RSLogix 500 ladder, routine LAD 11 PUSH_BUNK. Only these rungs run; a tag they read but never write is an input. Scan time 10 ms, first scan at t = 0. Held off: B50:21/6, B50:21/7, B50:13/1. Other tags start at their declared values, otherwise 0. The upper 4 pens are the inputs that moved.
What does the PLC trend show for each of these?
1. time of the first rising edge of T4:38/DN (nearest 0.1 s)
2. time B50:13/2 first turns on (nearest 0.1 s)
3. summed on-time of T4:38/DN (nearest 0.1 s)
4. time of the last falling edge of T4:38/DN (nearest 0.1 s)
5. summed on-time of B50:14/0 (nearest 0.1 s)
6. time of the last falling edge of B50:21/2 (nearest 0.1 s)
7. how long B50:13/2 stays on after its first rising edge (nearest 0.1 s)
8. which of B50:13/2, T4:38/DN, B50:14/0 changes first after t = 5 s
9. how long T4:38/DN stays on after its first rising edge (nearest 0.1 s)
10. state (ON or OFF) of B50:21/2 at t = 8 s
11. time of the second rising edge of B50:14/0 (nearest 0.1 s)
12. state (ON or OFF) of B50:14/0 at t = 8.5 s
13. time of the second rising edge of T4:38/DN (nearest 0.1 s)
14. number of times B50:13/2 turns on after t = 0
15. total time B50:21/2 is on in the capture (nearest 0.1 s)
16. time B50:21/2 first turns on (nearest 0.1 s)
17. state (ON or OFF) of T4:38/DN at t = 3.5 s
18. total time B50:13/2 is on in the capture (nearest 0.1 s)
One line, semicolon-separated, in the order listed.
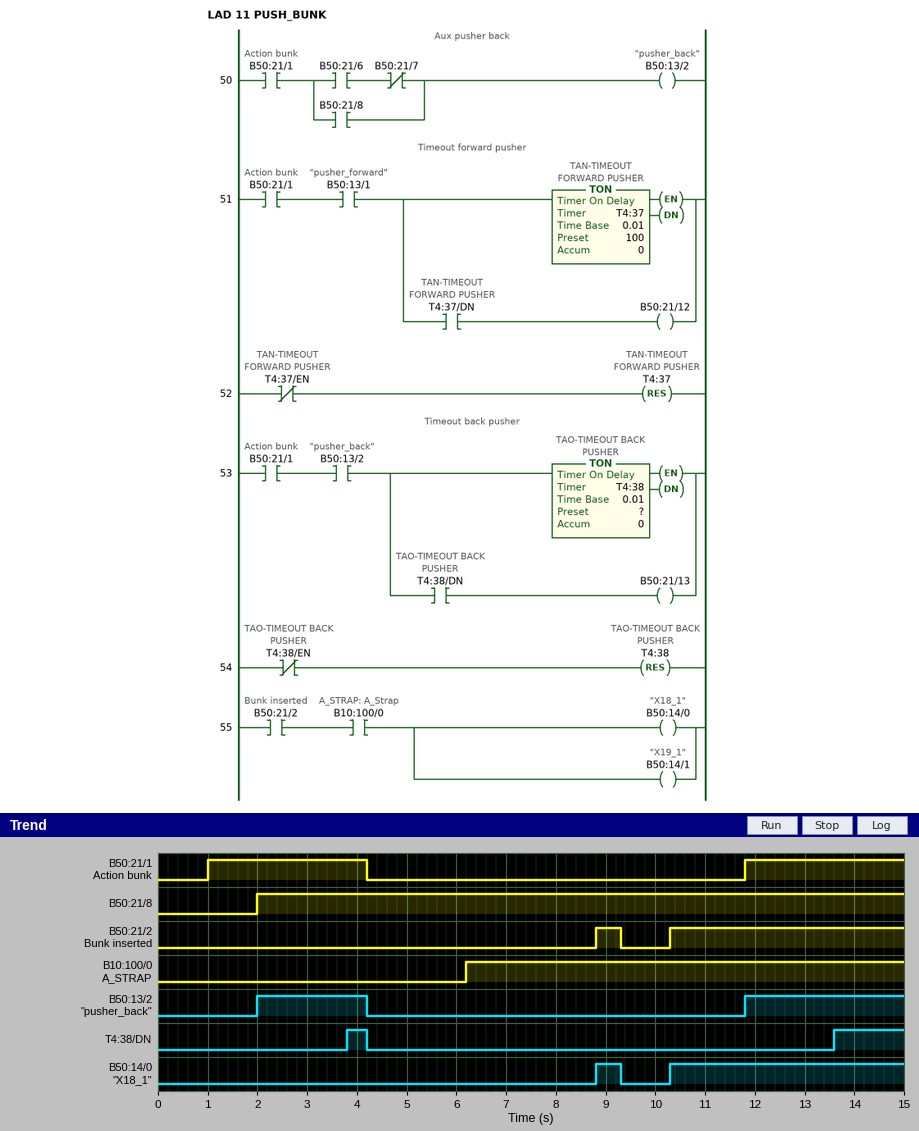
3.8 s; 2.0 s; 1.8 s; 4.2 s; 5.2 s; 9.3 s; 2.2 s; B50:14/0; 0.4 s; OFF; 10.3 s; OFF; 13.6 s; 2; 5.2 s; 8.8 s; OFF; 5.4 s
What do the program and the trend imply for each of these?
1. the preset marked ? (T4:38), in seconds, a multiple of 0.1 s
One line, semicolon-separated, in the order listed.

1.8 s
